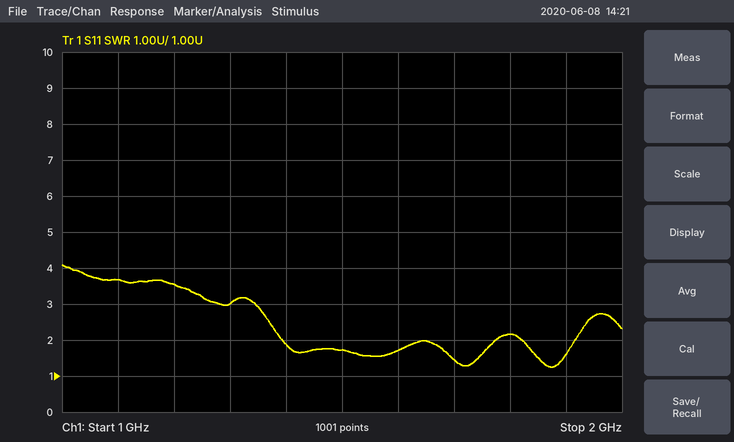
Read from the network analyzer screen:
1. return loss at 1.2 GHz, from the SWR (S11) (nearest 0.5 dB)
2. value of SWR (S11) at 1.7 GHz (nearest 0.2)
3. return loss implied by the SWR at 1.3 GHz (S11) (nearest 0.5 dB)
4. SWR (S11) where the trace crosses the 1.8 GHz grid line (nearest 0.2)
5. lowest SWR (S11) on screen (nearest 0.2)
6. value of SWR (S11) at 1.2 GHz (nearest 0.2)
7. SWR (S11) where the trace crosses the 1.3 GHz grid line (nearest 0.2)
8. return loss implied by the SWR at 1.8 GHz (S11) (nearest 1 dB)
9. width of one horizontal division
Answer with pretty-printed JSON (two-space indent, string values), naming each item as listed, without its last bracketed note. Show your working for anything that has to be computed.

{
  "return loss at 1.2 GHz, from the SWR (S11)": "−20 log10((3.6 − 1)/(3.6 + 1)) ≈ 5.0 dB",
  "value of SWR (S11) at 1.7 GHz": "1.4",
  "return loss implied by the SWR at 1.3 GHz (S11)": "−20 log10((3 − 1)/(3 + 1)) ≈ 6.0 dB",
  "SWR (S11) where the trace crosses the 1.8 GHz grid line": "2.2",
  "lowest SWR (S11) on screen": "1.2",
  "value of SWR (S11) at 1.2 GHz": "3.6",
  "SWR (S11) where the trace crosses the 1.3 GHz grid line": "3.0",
  "return loss implied by the SWR at 1.8 GHz (S11)": "−20 log10((2.2 − 1)/(2.2 + 1)) ≈ 9 dB",
  "width of one horizontal division": "100 MHz"
}
